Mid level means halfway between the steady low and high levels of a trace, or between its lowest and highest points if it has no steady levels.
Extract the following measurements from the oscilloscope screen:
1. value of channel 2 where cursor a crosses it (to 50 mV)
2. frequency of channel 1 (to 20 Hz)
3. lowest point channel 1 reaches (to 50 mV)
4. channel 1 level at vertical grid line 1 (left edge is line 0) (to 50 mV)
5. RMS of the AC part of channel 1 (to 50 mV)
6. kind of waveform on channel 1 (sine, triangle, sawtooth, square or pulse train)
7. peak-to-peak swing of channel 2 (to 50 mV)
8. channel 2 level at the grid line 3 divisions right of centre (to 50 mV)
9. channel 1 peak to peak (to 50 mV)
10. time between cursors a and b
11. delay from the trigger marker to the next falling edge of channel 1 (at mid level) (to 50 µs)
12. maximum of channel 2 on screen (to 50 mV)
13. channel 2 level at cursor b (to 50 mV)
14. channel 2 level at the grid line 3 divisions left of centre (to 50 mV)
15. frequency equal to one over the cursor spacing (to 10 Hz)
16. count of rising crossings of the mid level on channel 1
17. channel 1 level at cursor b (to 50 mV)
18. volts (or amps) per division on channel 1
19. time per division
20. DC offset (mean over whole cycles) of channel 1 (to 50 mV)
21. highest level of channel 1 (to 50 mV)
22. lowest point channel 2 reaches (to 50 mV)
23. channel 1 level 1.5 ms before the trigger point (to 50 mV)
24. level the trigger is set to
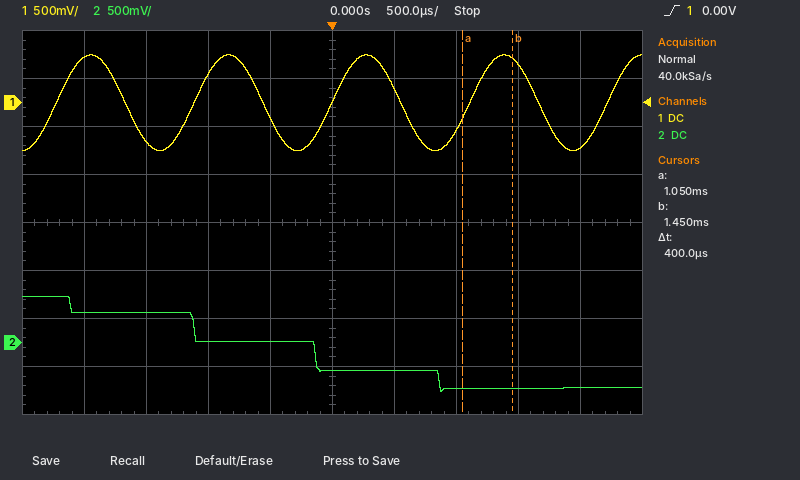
-500 mV
900 Hz
-500 mV
450 mV
350 mV
sine
1.00 V
-500 mV
1.00 V
400 µs
550 µs
500 mV
-500 mV
300 mV
2.50 kHz
5
450 mV
500 mV
500 µs
0 mV
500 mV
-500 mV
-400 mV
0.00 V
